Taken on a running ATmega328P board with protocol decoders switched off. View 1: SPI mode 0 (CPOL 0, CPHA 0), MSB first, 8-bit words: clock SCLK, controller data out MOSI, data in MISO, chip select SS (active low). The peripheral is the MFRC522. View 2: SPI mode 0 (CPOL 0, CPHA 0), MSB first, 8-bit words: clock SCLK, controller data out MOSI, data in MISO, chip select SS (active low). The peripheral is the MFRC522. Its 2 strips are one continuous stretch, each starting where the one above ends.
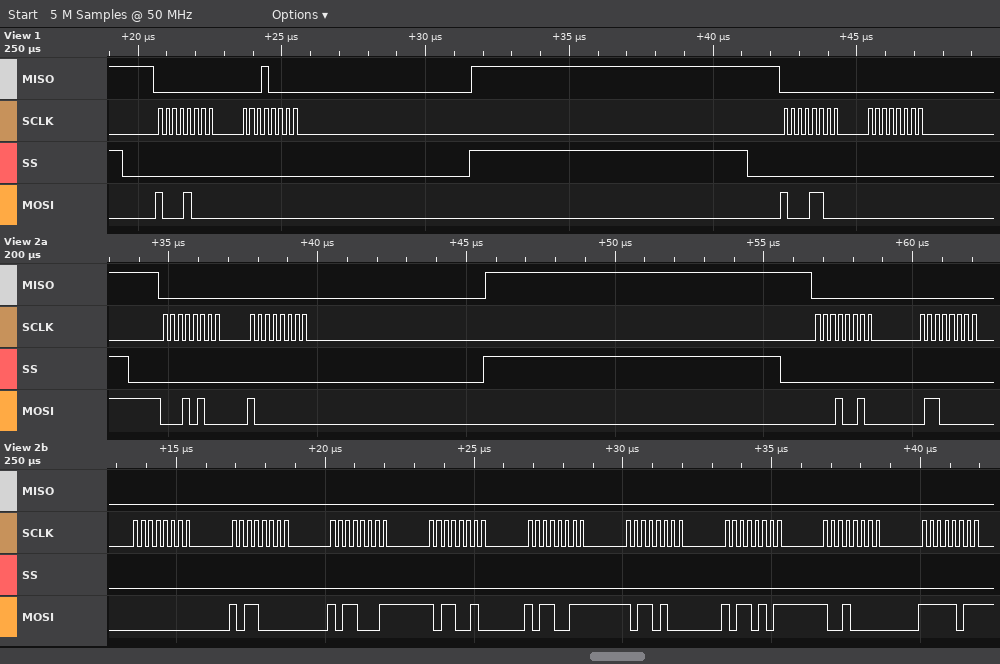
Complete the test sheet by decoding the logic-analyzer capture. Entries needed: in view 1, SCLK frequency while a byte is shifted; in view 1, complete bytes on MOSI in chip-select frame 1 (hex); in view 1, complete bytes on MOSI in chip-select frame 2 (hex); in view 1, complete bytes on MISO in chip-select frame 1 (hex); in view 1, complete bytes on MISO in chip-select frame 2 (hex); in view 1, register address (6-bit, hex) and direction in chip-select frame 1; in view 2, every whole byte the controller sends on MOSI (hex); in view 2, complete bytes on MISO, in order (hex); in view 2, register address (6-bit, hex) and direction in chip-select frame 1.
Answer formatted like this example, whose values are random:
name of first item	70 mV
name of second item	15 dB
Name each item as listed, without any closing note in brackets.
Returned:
in view 1, SCLK frequency while a byte is shifted	4 MHz
in view 1, complete bytes on MOSI in chip-select frame 1	0x88 0x00
in view 1, complete bytes on MOSI in chip-select frame 2	0x8C 0x00
in view 1, complete bytes on MISO in chip-select frame 1	0x00 0x10
in view 1, complete bytes on MISO in chip-select frame 2	0x00 0x00
in view 1, register address (6-bit, hex) and direction in chip-select frame 1	0x04 read
in view 2, every whole byte the controller sends on MOSI	14 80 12 60 00 B0 B1 B2 B3 B4 B5 90 FB
in view 2, complete bytes on MISO, in order	00 00 00 00 00 00 00 00 00 00 00 00 00
in view 2, register address (6-bit, hex) and direction in chip-select frame 1	0x0A write
